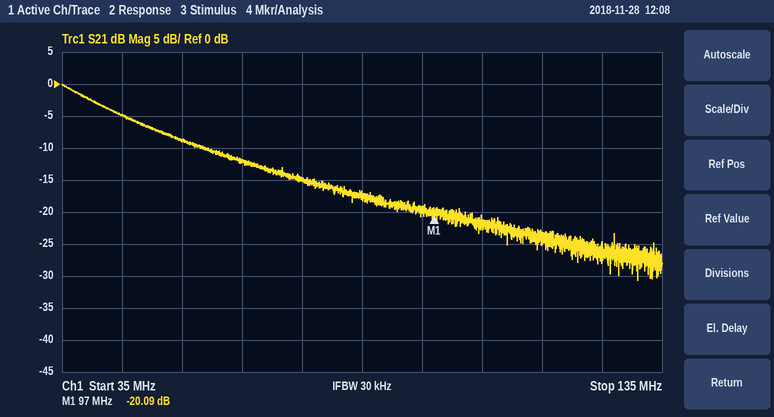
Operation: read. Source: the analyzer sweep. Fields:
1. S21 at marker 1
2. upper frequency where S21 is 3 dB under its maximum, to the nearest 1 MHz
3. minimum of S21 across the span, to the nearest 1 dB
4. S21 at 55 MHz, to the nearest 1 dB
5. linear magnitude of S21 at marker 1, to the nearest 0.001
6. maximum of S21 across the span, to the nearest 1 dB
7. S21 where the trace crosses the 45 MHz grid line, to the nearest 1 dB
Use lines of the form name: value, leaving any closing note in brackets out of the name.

S21 at marker 1: -20.09 dB
upper frequency where S21 is 3 dB under its maximum, to the nearest 1 MHz: 41 MHz
minimum of S21 across the span, to the nearest 1 dB: -31 dB
S21 at 55 MHz, to the nearest 1 dB: -9 dB
linear magnitude of S21 at marker 1, to the nearest 0.001: 0.099
maximum of S21 across the span, to the nearest 1 dB: 0 dB
S21 where the trace crosses the 45 MHz grid line, to the nearest 1 dB: -5 dB
